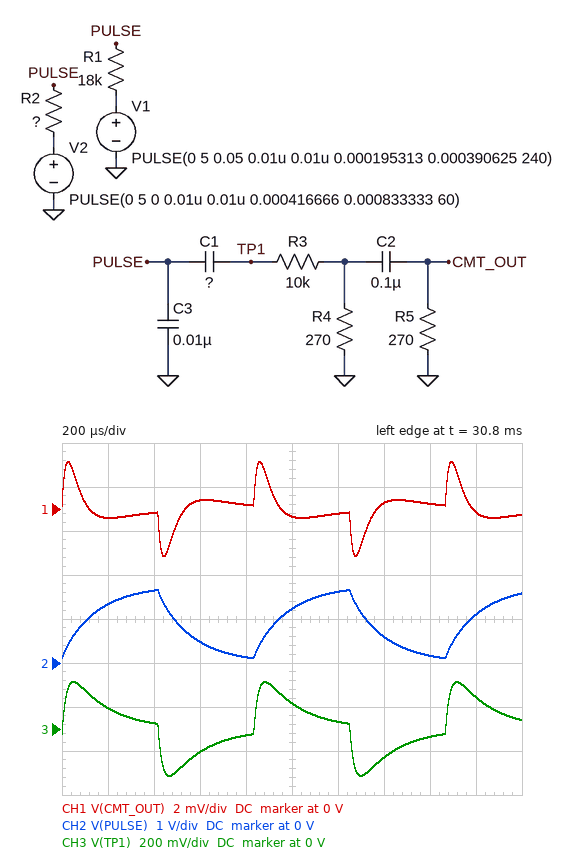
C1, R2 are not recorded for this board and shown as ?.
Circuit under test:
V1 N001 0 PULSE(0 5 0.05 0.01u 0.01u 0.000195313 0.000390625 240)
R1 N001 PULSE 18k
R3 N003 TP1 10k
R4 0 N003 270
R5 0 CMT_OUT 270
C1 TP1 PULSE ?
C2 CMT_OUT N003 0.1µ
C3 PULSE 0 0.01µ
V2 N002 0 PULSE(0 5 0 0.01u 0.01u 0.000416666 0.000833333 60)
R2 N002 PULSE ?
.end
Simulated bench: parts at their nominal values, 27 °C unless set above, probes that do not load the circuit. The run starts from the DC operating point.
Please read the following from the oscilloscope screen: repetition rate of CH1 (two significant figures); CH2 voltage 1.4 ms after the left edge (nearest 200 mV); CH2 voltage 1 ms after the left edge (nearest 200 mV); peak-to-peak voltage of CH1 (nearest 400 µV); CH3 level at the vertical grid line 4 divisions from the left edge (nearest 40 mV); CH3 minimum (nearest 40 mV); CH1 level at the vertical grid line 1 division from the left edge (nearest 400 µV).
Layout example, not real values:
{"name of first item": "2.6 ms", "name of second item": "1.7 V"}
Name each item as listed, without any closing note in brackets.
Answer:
{"repetition rate of CH1": "1.2 kHz", "CH2 voltage 1.4 ms after the left edge": "600 mV", "CH2 voltage 1 ms after the left edge": "1.2 V", "peak-to-peak voltage of CH1": "4.4 mV", "CH3 level at the vertical grid line 4 divisions from the left edge": "-40 mV", "CH3 minimum": "-200 mV", "CH1 level at the vertical grid line 1 division from the left edge": "-400 µV"}
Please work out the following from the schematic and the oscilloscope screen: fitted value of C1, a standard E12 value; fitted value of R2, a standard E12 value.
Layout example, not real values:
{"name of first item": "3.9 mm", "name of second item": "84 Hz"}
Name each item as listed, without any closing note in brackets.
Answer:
{"fitted value of C1, a standard E12 value": "2.7 nF", "fitted value of R2, a standard E12 value": "33 kΩ"}
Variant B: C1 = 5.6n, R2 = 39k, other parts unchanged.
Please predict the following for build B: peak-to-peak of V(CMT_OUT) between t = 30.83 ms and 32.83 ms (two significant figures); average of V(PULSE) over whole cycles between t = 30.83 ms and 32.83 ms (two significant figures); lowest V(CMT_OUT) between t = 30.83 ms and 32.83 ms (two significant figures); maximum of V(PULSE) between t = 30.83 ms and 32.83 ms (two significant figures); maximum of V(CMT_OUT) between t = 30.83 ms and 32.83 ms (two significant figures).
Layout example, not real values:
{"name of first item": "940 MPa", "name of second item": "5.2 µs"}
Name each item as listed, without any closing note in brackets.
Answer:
{"peak-to-peak of V(CMT_OUT) between t = 30.83 ms and 32.83 ms": "5.0 mV", "average of V(PULSE) over whole cycles between t = 30.83 ms and 32.83 ms": "790 mV", "lowest V(CMT_OUT) between t = 30.83 ms and 32.83 ms": "-2.5 mV", "maximum of V(PULSE) between t = 30.83 ms and 32.83 ms": "1.4 V", "maximum of V(CMT_OUT) between t = 30.83 ms and 32.83 ms": "2.5 mV"}
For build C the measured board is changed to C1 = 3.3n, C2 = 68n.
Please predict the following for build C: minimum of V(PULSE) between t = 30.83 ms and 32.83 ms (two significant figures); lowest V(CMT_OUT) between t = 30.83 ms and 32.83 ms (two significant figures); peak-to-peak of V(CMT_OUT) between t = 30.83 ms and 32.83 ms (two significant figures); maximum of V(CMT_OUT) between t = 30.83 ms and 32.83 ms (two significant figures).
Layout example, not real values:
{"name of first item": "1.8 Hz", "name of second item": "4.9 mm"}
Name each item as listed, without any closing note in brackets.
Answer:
{"minimum of V(PULSE) between t = 30.83 ms and 32.83 ms": "120 mV", "lowest V(CMT_OUT) between t = 30.83 ms and 32.83 ms": "-2.0 mV", "peak-to-peak of V(CMT_OUT) between t = 30.83 ms and 32.83 ms": "4.0 mV", "maximum of V(CMT_OUT) between t = 30.83 ms and 32.83 ms": "2.0 mV"}
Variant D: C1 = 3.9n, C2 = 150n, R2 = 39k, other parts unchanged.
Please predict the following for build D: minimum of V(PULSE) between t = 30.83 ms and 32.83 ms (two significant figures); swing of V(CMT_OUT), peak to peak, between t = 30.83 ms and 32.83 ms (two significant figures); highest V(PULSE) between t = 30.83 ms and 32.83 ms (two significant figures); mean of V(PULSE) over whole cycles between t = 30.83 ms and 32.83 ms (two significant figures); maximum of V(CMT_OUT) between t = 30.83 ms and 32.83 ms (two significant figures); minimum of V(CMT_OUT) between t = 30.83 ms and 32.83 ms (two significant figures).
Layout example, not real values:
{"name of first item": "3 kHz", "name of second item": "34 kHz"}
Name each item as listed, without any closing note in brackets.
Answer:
{"minimum of V(PULSE) between t = 30.83 ms and 32.83 ms": "140 mV", "swing of V(CMT_OUT), peak to peak, between t = 30.83 ms and 32.83 ms": "5.1 mV", "highest V(PULSE) between t = 30.83 ms and 32.83 ms": "1.4 V", "mean of V(PULSE) over whole cycles between t = 30.83 ms and 32.83 ms": "790 mV", "maximum of V(CMT_OUT) between t = 30.83 ms and 32.83 ms": "2.5 mV", "minimum of V(CMT_OUT) between t = 30.83 ms and 32.83 ms": "-2.5 mV"}
